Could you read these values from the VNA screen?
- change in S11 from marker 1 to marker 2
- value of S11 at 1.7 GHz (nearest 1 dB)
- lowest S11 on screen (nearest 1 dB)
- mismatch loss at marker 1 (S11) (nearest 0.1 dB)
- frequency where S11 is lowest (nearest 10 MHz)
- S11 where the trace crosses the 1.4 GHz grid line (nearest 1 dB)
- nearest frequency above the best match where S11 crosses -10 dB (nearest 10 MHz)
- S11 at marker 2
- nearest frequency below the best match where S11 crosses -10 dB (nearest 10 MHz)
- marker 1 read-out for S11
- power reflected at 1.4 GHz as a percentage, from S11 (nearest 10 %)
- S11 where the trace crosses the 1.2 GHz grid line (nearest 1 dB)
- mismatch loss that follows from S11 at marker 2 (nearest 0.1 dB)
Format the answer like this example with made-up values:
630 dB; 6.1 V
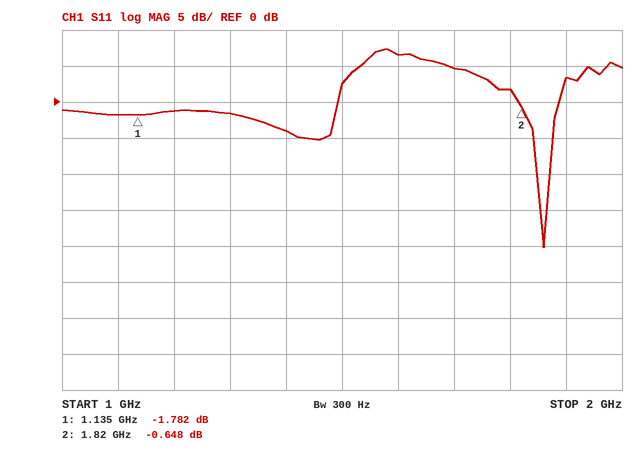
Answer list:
1.134 dB; 5 dB; -20 dB; 4.7 dB; 1.86 GHz; -4 dB; 1.87 GHz; -0.648 dB; 1.85 GHz; -1.782 dB; 40 %; -1 dB; 8.6 dB
